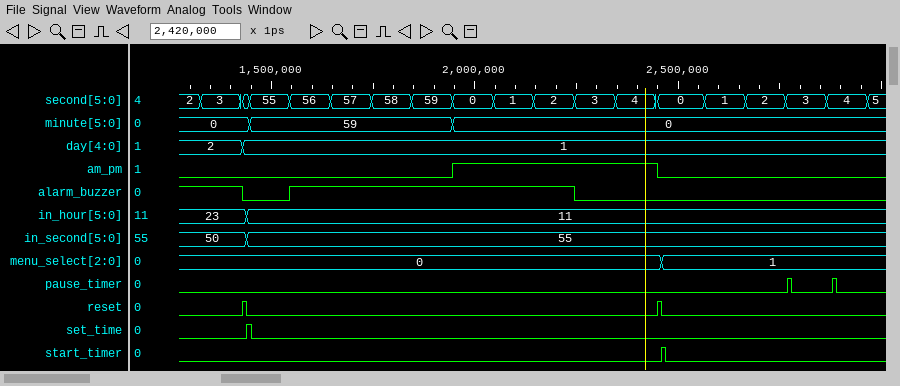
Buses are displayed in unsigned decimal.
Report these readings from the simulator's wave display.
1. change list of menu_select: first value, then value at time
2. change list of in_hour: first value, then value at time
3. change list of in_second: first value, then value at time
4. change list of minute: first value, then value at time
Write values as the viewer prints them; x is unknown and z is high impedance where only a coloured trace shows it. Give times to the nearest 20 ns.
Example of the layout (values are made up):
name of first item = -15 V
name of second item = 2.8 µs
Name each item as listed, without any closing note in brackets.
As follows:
change list of menu_select: first value, then value at time = 0, 1 at 2460 ns
change list of in_hour: first value, then value at time = 23, 11 at 1440 ns
change list of in_second: first value, then value at time = 50, 55 at 1440 ns
change list of minute: first value, then value at time = 0, 59 at 1440 ns, 0 at 1940 ns
